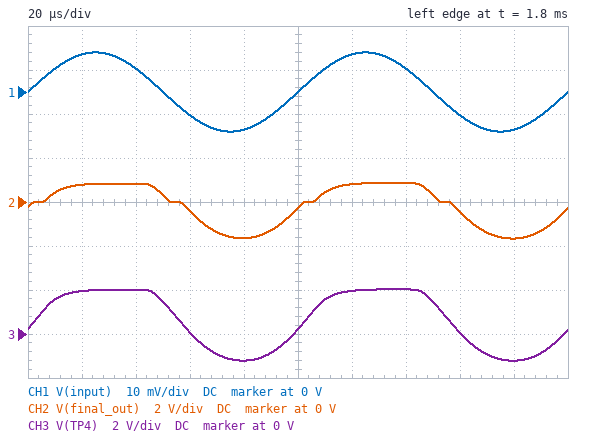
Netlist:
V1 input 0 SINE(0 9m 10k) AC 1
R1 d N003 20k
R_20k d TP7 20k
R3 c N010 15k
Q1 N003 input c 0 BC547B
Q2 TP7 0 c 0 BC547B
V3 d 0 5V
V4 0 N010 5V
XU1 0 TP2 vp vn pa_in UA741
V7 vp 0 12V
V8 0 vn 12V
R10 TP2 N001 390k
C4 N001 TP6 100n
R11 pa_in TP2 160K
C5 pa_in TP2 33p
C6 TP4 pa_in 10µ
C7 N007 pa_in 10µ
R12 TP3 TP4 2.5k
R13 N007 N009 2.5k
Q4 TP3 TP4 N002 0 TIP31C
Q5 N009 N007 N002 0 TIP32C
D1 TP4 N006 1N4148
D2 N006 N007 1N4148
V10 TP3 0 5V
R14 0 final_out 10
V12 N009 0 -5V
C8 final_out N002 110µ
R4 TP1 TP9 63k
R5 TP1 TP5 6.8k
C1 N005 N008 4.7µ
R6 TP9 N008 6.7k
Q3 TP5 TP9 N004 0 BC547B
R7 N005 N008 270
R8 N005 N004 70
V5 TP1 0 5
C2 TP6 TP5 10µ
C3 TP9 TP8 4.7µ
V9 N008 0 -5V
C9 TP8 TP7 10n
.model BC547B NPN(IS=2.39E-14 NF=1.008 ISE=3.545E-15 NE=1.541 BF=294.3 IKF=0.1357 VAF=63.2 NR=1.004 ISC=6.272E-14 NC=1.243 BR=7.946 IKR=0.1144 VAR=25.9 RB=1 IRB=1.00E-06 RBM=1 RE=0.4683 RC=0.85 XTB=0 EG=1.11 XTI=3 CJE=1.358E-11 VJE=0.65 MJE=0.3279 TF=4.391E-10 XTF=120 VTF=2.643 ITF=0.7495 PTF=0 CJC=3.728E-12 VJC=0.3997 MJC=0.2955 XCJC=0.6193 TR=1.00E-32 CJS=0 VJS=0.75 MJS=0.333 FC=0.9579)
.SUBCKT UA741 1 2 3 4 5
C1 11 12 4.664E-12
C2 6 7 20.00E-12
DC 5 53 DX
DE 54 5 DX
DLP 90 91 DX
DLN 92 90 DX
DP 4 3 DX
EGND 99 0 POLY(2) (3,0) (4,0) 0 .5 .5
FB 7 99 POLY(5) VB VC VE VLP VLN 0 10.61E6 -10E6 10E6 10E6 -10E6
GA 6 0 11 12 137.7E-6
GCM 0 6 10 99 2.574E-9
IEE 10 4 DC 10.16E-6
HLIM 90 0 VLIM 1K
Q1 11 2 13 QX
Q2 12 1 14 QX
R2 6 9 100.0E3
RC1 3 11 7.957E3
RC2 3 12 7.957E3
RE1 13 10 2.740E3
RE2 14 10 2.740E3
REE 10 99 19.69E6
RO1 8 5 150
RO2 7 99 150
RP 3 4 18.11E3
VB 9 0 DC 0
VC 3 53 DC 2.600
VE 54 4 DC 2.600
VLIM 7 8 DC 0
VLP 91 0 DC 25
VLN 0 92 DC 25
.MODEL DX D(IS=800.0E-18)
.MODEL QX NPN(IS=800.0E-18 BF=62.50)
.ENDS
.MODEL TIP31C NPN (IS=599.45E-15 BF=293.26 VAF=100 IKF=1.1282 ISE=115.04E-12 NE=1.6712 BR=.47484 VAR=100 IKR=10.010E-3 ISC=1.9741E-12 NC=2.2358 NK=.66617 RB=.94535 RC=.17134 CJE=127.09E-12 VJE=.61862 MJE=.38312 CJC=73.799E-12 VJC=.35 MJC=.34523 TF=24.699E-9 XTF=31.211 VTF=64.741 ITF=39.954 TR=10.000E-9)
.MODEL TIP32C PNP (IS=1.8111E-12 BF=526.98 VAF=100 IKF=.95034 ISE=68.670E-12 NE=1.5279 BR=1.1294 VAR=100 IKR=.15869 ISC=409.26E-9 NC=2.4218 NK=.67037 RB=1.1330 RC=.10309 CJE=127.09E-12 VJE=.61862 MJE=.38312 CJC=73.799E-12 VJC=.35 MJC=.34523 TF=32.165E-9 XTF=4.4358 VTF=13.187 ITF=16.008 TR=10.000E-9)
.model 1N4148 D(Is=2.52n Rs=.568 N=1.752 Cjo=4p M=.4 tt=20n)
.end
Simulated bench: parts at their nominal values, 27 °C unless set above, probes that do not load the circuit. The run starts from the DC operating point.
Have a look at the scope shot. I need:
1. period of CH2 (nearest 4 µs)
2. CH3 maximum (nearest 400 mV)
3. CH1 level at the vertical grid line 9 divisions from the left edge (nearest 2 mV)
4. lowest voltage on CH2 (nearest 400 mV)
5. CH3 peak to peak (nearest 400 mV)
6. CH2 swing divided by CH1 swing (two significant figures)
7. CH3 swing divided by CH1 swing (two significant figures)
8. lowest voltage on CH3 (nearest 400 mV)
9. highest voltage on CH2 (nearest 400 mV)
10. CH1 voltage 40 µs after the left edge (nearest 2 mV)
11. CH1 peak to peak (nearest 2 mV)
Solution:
100 µs
2.0 V
-8 mV
-1.6 V
3.2 V
140
180
-1.2 V
800 mV
6 mV
18 mV
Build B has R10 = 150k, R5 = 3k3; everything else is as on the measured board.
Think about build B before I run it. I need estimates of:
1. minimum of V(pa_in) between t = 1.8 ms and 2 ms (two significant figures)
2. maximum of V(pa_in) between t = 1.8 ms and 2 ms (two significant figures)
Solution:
-4.6 V
1.1 V
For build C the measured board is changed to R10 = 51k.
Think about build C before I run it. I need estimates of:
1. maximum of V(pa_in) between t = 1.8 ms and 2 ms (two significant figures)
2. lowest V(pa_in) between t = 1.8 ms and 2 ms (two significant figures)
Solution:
7.6 V
-5.2 V
